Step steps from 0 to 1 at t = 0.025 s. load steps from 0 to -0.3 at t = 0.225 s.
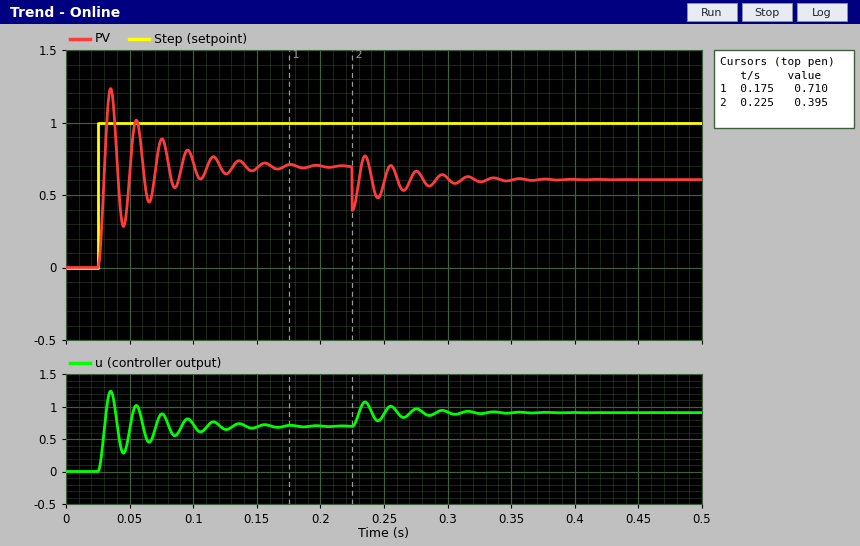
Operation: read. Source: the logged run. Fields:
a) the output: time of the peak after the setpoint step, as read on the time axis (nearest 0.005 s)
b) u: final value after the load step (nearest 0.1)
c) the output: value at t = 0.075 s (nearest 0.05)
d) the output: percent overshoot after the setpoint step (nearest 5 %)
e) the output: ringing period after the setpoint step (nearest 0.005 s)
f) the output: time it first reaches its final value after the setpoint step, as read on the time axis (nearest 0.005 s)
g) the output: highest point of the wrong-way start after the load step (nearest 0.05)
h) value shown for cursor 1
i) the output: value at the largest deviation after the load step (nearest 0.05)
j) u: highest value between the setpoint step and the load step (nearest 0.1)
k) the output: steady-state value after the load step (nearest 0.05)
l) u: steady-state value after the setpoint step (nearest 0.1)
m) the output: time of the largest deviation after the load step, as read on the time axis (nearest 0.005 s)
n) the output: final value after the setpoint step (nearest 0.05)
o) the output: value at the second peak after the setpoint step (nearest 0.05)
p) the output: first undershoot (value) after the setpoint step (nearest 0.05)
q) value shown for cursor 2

0.035 s
0.9
0.90
75 %
0.020 s
0.030 s
0.75
0.710
0.40
1.2
0.60
0.7
0.225 s
0.70
1.00
0.30
0.395
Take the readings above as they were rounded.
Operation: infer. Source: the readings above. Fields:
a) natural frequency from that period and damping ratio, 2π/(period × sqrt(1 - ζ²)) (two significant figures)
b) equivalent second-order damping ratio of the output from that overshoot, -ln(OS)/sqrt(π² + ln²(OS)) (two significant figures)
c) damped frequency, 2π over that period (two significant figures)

320 rad/s
0.091
310 rad/s
